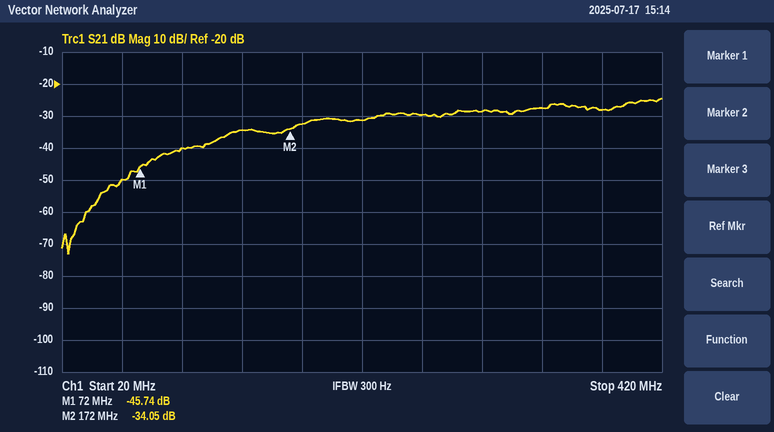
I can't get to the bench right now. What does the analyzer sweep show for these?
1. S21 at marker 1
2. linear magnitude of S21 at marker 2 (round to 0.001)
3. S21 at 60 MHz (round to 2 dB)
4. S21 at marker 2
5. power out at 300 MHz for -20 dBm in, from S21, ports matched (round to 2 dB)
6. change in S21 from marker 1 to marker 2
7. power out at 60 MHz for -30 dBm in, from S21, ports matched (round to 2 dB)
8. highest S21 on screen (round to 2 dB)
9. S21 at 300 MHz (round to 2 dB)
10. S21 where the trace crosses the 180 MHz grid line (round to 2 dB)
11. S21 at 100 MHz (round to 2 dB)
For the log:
-45.74 dB
0.020
-50 dB
-34.05 dB
-48 dBm
11.69 dB
-80 dBm
-24 dB
-28 dB
-32 dB
-40 dB
